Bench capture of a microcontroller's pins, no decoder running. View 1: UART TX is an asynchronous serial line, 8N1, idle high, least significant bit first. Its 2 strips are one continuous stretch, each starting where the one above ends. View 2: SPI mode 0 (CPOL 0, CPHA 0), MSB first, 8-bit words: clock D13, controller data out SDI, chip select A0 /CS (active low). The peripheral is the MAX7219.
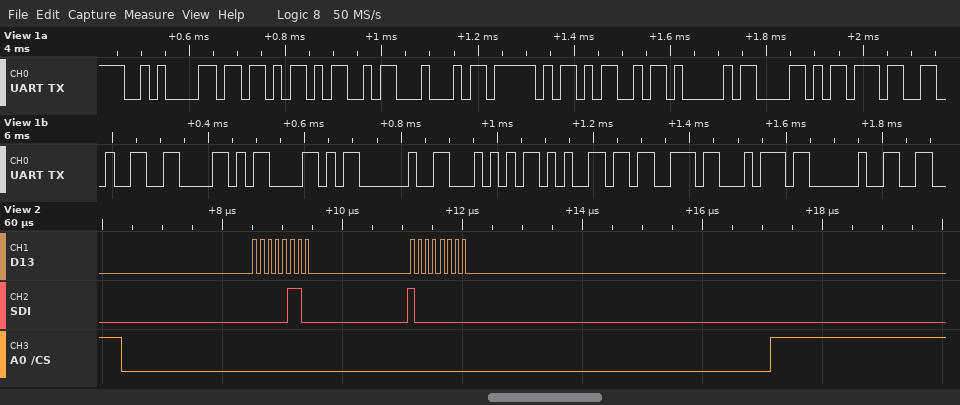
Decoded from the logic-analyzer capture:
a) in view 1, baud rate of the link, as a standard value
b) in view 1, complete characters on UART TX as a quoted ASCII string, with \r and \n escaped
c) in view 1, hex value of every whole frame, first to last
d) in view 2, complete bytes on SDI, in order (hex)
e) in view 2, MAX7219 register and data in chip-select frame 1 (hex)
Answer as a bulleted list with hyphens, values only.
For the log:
- 57600 baud
- "\n[MD_MAX72XX Test "
- 0A 5B 4D 44 5F 4D 41 58 37 32 58 58 20 54 65 73 74 20
- 06 80
- register 0x6, data 0x80
